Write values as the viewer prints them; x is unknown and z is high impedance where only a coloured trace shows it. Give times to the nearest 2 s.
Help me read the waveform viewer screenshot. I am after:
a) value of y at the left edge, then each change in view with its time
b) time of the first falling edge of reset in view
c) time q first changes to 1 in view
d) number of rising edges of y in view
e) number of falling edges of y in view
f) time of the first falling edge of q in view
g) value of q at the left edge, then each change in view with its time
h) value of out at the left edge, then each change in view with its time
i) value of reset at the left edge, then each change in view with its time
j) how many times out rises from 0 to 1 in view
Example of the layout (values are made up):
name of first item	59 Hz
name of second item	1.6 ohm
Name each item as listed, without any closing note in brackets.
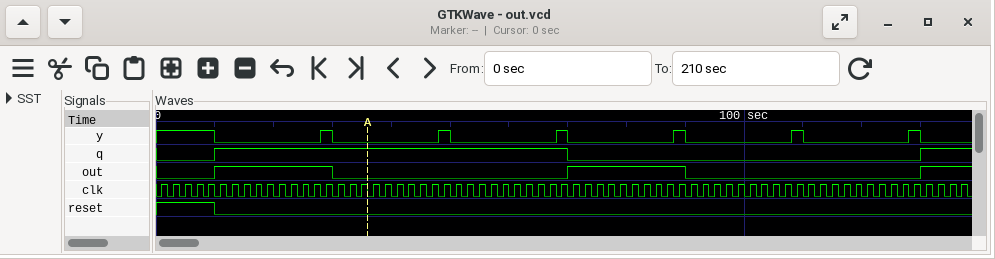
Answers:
value of y at the left edge, then each change in view with its time	1, 0 at 10 s, 1 at 28 s, 0 at 30 s, 1 at 48 s, 0 at 50 s, 1 at 68 s, 0 at 70 s, 1 at 88 s, 0 at 90 s, 1 at 108 s, 0 at 110 s, 1 at 128 s, 0 at 130 s
time of the first falling edge of reset in view	10 s
time q first changes to 1 in view	10 s
number of rising edges of y in view	6
number of falling edges of y in view	7
time of the first falling edge of q in view	70 s
value of q at the left edge, then each change in view with its time	0, 1 at 10 s, 0 at 70 s, 1 at 130 s
value of out at the left edge, then each change in view with its time	0, 1 at 10 s, 0 at 30 s, 1 at 70 s, 0 at 90 s, 1 at 130 s
value of reset at the left edge, then each change in view with its time	1, 0 at 10 s
how many times out rises from 0 to 1 in view	3
